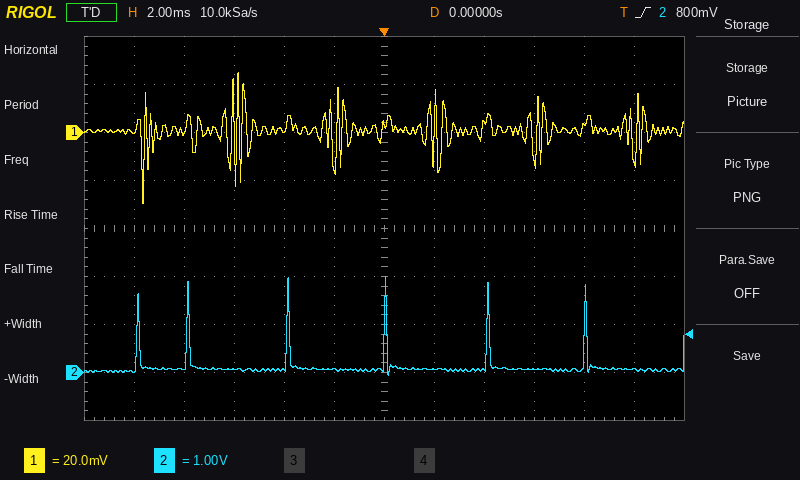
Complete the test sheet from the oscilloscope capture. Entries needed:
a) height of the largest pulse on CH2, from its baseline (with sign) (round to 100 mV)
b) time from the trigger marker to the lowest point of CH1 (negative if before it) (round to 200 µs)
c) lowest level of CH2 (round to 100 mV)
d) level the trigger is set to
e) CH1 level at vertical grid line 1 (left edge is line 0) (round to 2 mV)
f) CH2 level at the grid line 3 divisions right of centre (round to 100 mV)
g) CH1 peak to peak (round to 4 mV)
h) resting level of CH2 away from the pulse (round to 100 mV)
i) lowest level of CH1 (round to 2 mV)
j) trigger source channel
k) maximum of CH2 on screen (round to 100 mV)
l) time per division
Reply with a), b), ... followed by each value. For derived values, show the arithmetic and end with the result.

a) 2.0 V − (100 mV) = +1.9 V
b) -9.6 ms
c) -100 mV
d) 800 mV
e) 2 mV
f) 100 mV
g) 56 mV
h) 100 mV
i) -30 mV
j) CH2
k) 2.0 V
l) 2 ms
